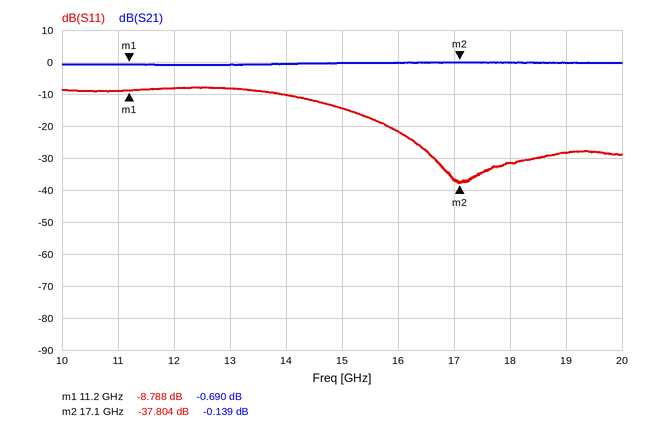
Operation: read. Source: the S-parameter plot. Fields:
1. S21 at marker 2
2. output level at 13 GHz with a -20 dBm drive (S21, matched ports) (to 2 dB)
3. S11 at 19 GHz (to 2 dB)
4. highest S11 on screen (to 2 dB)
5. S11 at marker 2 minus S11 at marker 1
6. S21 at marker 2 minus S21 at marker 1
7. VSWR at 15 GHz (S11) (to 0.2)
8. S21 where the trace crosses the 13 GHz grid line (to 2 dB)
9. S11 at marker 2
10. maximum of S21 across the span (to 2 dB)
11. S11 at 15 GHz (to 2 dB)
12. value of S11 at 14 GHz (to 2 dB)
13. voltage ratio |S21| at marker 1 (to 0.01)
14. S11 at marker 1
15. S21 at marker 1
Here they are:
-0.139 dB
-20 dBm
-28 dB
-8 dB
-29.016 dB
0.551 dB
1.4
0 dB
-37.804 dB
0 dB
-14 dB
-10 dB
0.92
-8.788 dB
-0.690 dB
